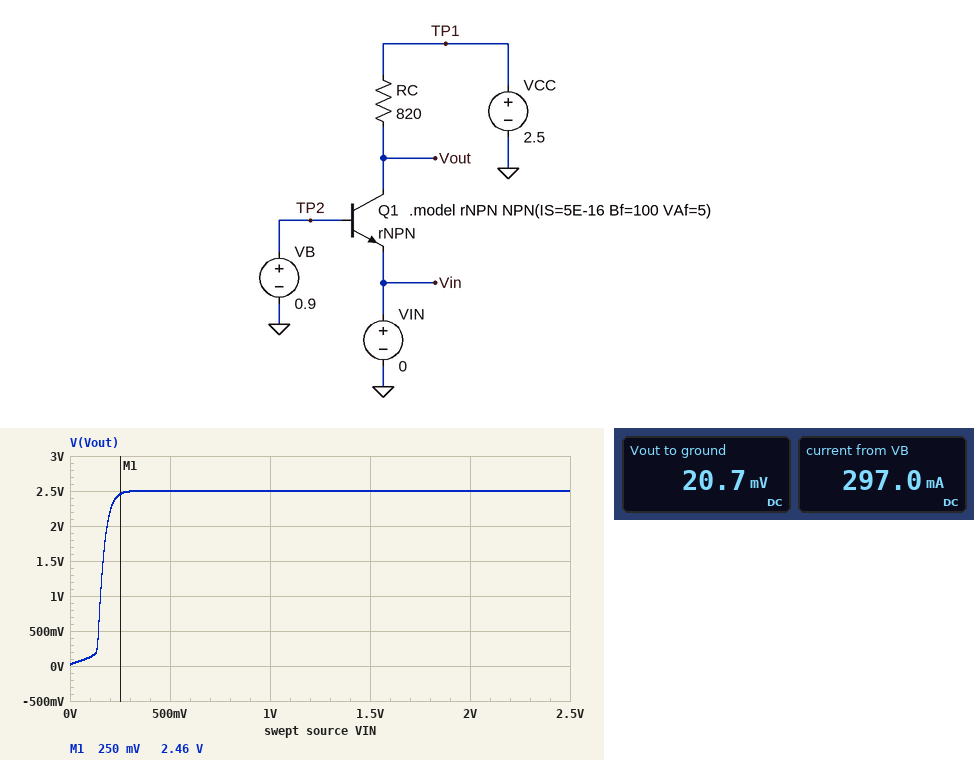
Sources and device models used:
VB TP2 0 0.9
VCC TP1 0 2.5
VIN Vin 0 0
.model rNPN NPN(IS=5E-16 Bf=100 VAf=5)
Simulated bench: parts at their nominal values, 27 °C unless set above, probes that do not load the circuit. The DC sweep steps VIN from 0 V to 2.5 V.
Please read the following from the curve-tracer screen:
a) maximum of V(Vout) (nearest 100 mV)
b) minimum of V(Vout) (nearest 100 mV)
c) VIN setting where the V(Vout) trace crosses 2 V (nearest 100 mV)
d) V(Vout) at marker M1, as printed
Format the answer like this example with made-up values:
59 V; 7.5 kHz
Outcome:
2.5 V; 0 V; 200 mV; 2.46 V
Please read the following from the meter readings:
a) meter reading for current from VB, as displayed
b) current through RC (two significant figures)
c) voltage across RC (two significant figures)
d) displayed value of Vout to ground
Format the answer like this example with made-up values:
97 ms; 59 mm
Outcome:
297.0 mA; 3.0 mA; 2.5 V; 20.7 mV
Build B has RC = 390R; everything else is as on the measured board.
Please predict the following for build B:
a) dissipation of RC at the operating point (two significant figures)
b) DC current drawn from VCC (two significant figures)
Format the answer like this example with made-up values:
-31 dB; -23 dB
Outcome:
16 mW; 6.4 mA
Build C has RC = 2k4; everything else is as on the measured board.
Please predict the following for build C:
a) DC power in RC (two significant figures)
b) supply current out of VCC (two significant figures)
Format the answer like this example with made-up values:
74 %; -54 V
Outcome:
2.6 mW; 1.0 mA
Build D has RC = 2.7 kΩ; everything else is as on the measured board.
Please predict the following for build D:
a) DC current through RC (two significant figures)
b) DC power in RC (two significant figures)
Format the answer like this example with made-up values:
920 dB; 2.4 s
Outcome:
920 µA; 2.3 mW
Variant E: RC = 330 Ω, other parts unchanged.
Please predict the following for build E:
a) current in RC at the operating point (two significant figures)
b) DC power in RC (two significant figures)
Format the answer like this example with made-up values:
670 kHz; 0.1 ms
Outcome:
7.5 mA; 19 mW
